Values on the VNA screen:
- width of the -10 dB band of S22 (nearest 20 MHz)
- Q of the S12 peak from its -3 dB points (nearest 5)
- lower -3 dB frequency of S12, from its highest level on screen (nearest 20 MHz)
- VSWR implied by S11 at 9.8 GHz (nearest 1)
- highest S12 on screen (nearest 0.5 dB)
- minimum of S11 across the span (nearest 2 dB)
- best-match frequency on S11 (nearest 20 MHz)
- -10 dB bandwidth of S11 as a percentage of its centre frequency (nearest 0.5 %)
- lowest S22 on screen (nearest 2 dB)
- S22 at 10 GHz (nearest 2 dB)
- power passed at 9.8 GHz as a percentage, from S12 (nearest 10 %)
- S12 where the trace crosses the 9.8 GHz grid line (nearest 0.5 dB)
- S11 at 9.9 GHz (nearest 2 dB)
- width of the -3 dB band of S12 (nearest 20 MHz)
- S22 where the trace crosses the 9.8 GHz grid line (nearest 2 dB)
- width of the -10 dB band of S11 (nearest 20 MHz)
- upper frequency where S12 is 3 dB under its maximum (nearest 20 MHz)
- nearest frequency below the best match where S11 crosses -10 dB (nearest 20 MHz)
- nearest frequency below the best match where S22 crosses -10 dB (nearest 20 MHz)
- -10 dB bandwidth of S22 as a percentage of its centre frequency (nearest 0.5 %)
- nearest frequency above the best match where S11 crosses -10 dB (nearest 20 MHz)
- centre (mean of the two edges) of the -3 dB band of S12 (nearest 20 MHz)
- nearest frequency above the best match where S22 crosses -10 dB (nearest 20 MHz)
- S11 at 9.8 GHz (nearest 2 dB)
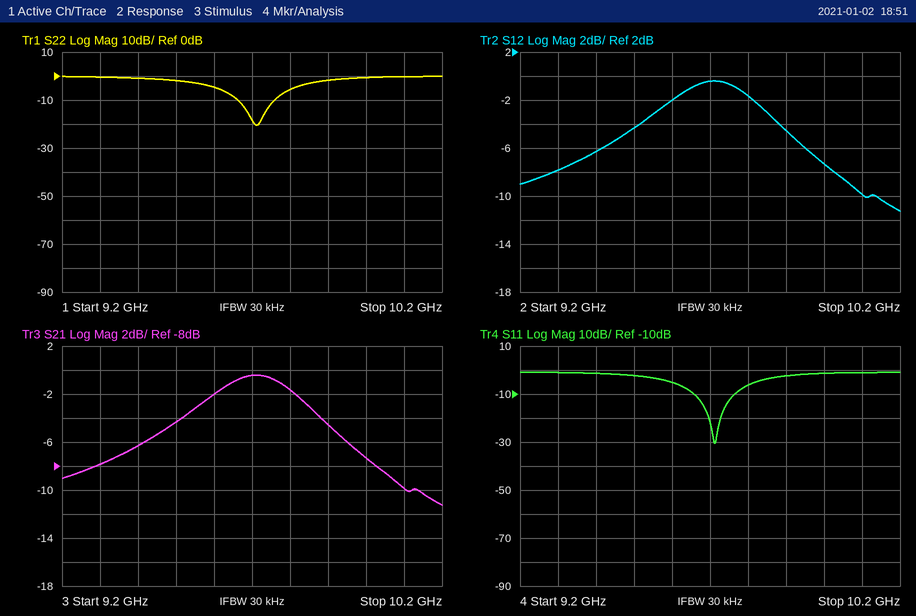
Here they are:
100 MHz
30
9.54 GHz
3
-0.5 dB
-30 dB
9.72 GHz
1.0 %
-20 dB
0 dB
70 %
-1.5 dB
-2 dB
320 MHz
-6 dB
100 MHz
9.86 GHz
9.66 GHz
9.66 GHz
1.0 %
9.76 GHz
9.70 GHz
9.76 GHz
-6 dB
